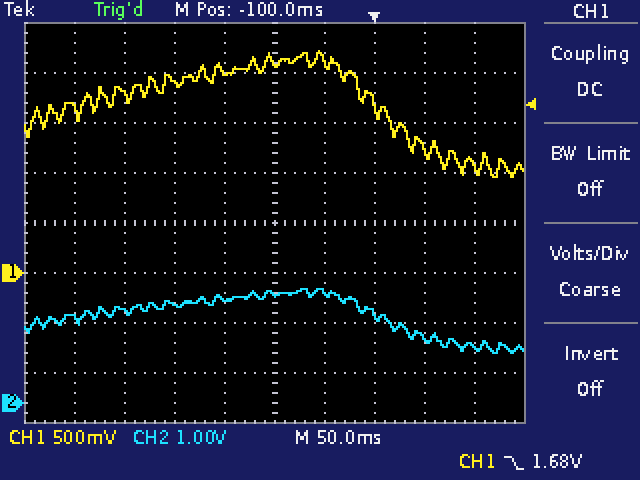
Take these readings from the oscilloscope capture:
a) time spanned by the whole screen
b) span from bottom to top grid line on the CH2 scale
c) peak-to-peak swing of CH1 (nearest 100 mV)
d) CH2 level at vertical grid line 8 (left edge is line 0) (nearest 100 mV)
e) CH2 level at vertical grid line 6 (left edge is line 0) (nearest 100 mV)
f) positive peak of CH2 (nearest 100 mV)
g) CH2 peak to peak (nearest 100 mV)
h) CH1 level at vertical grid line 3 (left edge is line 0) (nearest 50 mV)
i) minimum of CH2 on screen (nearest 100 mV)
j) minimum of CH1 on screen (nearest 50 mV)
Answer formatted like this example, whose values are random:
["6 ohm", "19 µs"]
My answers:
["500 ms", "8 V", "1.30 V", "1.3 V", "2.2 V", "2.3 V", "1.3 V", "1.90 V", "1.0 V", "950 mV"]
